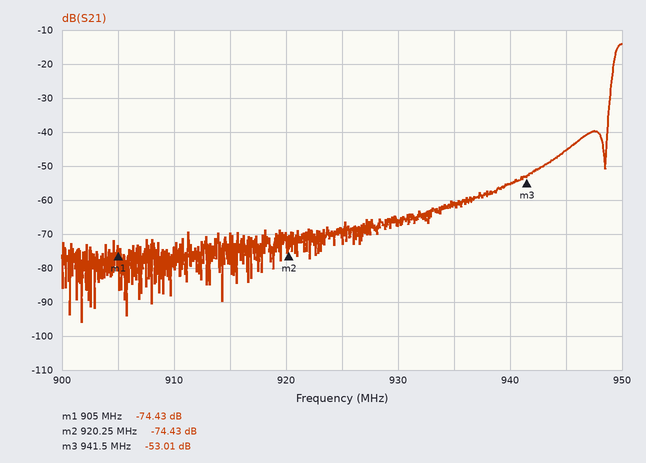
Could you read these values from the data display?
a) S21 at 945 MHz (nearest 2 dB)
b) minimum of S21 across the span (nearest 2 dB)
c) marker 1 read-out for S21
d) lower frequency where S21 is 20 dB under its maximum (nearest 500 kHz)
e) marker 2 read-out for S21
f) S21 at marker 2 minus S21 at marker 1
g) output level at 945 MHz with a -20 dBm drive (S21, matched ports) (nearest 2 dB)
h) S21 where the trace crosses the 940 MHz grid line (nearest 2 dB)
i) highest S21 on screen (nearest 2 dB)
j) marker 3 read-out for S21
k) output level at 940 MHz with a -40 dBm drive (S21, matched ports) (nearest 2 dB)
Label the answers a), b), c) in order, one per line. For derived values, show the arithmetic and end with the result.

a) -46 dB
b) -96 dB
c) -74.43 dB
d) 949.0 MHz
e) -74.43 dB
f) -74.43 − (-74.43) = 0.00 dB
g) -20 dBm + (-46 dB) = -66 dBm
h) -56 dB
i) -14 dB
j) -53.01 dB
k) -40 dBm + (-56 dB) = -96 dBm
